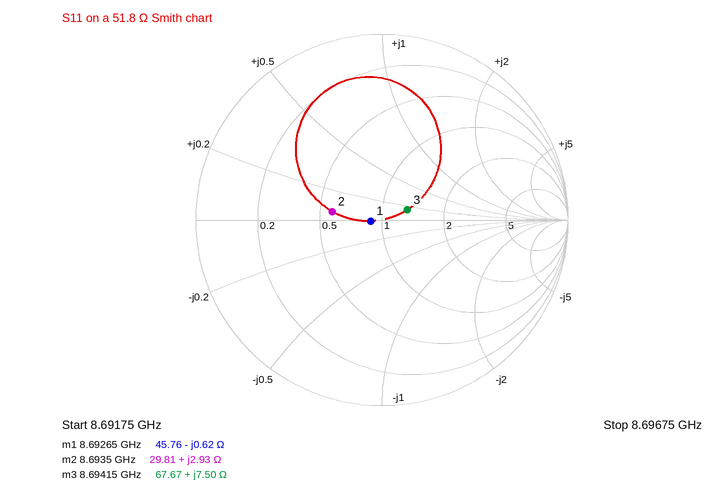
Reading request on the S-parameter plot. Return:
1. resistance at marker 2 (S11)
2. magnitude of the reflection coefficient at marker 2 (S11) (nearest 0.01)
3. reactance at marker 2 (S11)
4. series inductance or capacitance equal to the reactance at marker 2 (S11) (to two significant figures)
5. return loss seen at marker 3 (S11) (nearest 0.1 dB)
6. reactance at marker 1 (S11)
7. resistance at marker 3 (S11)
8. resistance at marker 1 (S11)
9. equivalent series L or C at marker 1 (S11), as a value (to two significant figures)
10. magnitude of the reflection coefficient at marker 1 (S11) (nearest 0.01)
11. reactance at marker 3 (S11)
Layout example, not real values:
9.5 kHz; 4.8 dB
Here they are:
29.81 Ω; 0.27; +2.93 Ω; 54 pH; 16.7 dB; -0.62 Ω; 67.67 Ω; 45.76 Ω; 30 pF; 0.06; +7.50 Ω
